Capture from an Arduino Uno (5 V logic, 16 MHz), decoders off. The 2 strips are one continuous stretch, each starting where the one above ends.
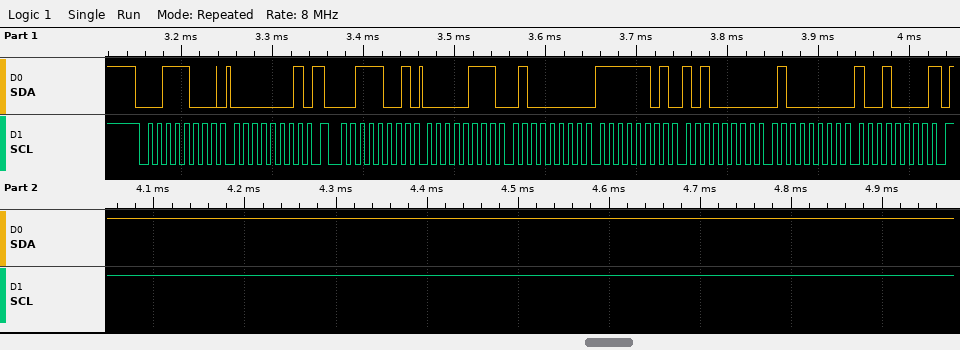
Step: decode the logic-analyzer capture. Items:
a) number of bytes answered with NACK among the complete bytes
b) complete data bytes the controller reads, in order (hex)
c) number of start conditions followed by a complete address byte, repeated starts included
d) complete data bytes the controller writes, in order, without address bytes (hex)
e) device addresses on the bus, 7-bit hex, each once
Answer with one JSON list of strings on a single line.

["1", "07 40 FD A0 40 90", "2", "01", "0x1C"]
